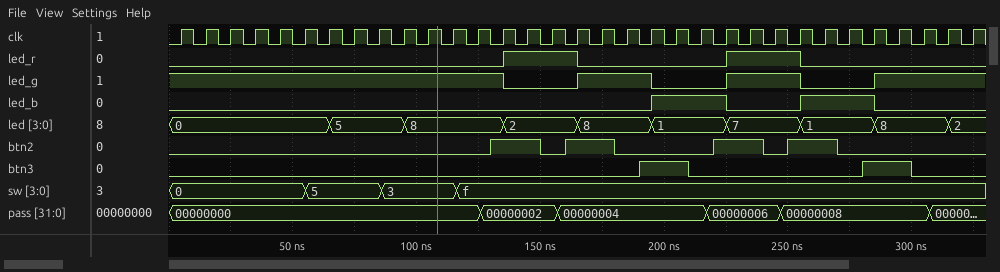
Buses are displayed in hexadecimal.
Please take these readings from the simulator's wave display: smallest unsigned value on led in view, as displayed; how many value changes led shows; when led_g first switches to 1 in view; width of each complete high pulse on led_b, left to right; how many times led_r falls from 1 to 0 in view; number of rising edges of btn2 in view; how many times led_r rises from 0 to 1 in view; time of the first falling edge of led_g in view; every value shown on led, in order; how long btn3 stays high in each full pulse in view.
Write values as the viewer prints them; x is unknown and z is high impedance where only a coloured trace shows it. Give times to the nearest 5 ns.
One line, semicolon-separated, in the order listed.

0; 9; 165 ns; 30 ns, 30 ns; 2; 4; 2; 135 ns; 0, 5, 8, 2, 8, 1, 7, 1, 8, 2; 20 ns, 20 ns
